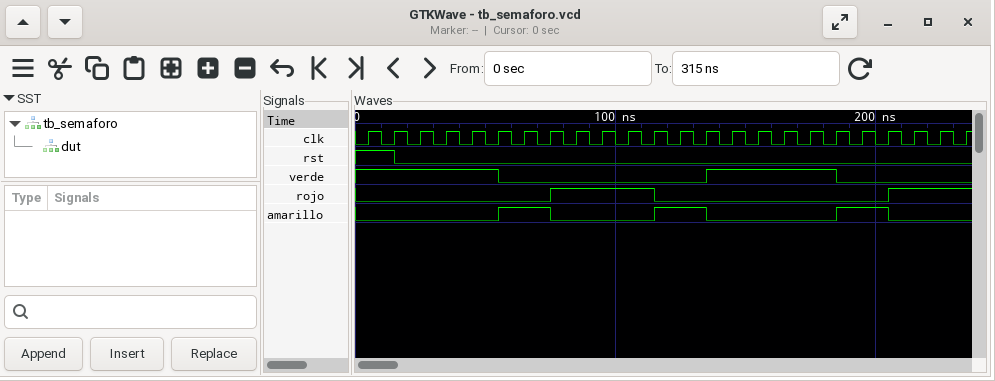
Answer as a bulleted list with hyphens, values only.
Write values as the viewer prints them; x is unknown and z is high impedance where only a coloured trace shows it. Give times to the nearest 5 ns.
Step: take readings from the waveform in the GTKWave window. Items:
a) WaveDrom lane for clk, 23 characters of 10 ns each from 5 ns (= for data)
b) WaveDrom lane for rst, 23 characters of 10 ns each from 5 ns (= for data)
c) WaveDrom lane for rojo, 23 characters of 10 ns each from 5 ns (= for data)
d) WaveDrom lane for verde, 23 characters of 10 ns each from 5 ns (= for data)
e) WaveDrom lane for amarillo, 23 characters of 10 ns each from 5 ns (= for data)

- {name: 'clk', wave: 'p......................'}
- {name: 'rst', wave: '10.....................'}
- {name: 'rojo', wave: '0......1...0........1..'}
- {name: 'verde', wave: '1....0.......1....0....'}
- {name: 'amarillo', wave: '0....1.0...1.0....1.0..'}
